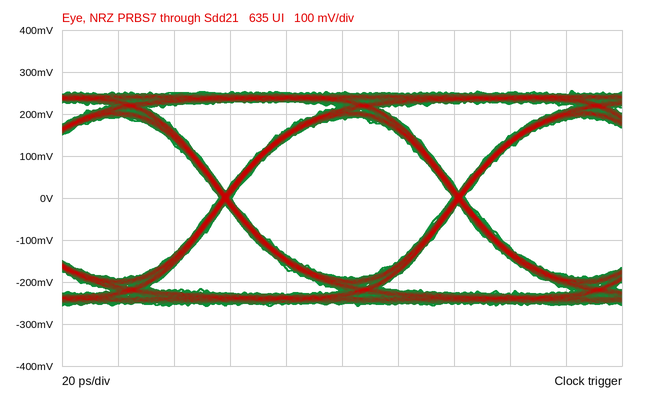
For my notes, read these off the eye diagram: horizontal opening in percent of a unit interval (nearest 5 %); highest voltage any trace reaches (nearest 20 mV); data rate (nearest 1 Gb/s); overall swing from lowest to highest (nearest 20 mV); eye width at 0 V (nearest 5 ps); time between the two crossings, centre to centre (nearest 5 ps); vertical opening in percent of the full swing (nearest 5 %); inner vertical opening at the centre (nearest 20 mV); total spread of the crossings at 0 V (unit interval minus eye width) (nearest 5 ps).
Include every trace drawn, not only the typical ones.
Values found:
95 %
260 mV
12 Gb/s
520 mV
80 ps
85 ps
75 %
380 mV
5 ps
